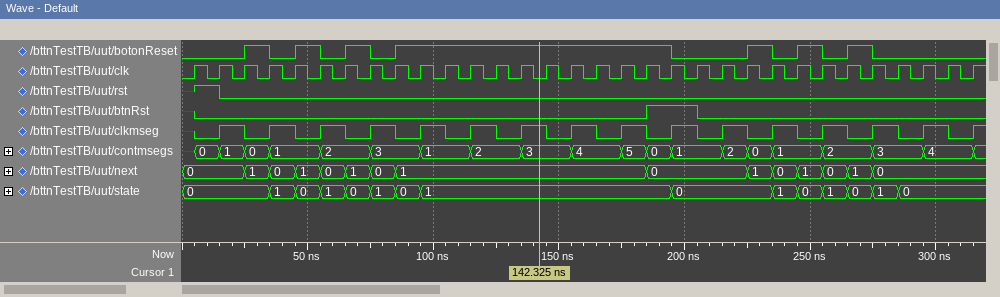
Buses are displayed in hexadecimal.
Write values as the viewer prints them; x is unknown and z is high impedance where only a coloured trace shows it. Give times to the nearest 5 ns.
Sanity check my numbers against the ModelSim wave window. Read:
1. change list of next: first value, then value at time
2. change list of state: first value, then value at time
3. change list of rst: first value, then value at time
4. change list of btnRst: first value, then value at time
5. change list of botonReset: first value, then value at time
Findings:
0, 1 at 25 ns, 0 at 35 ns, 1 at 45 ns, 0 at 55 ns, 1 at 65 ns, 0 at 75 ns, 1 at 85 ns, 0 at 185 ns, 1 at 225 ns, 0 at 235 ns, 1 at 245 ns, 0 at 255 ns, 1 at 265 ns, 0 at 275 ns
0, 1 at 35 ns, 0 at 45 ns, 1 at 55 ns, 0 at 65 ns, 1 at 75 ns, 0 at 85 ns, 1 at 95 ns, 0 at 195 ns, 1 at 235 ns, 0 at 245 ns, 1 at 255 ns, 0 at 265 ns, 1 at 275 ns, 0 at 285 ns
x, 1 at 5 ns, 0 at 15 ns
x, 0 at 5 ns, 1 at 185 ns, 0 at 205 ns
0, 1 at 25 ns, 0 at 35 ns, 1 at 45 ns, 0 at 55 ns, 1 at 65 ns, 0 at 75 ns, 1 at 85 ns, 0 at 195 ns, 1 at 225 ns, 0 at 235 ns, 1 at 245 ns, 0 at 255 ns, 1 at 265 ns, 0 at 275 ns
